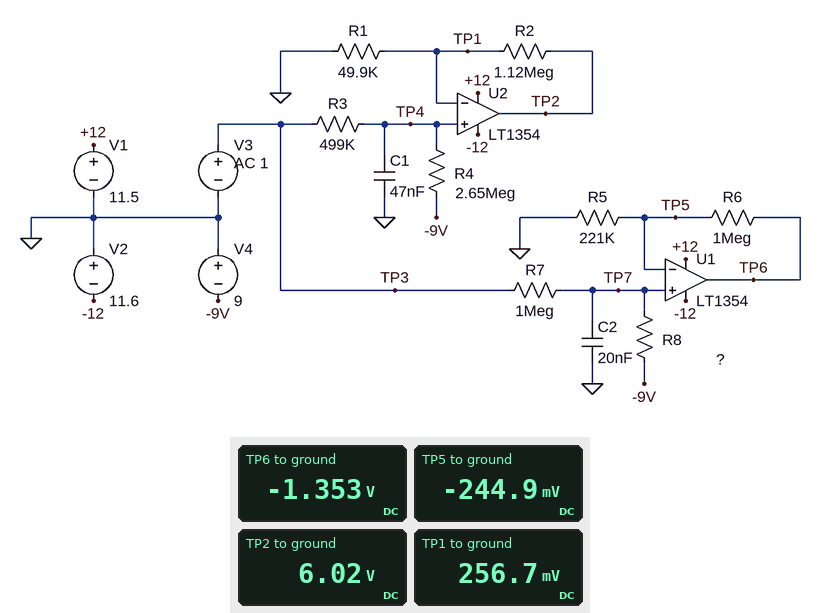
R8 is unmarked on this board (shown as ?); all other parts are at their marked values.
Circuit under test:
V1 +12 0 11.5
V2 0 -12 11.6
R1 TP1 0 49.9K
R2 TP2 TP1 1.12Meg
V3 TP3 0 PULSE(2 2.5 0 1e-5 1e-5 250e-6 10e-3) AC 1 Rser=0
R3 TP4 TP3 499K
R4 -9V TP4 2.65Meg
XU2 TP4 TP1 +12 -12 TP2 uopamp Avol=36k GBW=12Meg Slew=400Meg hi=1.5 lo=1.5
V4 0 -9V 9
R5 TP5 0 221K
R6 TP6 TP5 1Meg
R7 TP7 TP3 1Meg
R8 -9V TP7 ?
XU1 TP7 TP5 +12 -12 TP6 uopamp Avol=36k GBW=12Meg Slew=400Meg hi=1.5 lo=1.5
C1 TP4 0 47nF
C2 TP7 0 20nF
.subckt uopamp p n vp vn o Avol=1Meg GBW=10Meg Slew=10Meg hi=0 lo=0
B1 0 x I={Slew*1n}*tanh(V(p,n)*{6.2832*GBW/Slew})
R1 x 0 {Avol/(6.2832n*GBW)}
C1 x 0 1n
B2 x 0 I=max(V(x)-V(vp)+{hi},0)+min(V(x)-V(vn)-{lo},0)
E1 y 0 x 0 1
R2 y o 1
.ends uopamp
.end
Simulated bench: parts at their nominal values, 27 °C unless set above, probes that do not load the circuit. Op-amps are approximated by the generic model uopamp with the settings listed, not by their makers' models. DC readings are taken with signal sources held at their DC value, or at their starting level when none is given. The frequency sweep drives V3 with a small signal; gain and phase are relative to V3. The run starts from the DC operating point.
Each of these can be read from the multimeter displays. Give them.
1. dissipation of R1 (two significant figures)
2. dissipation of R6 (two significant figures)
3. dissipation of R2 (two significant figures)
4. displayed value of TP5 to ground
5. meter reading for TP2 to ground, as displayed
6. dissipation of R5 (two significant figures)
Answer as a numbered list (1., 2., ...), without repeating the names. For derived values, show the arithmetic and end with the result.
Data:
1. (256.7 mV)^2 / 49.9 kΩ = 1.3 µW
2. (-244.9 mV - (-1.353 V))^2 / 1 MΩ = 1.2 µW
3. (6.02 V - 256.7 mV)^2 / 1.12 MΩ = 30 µW
4. -244.9 mV
5. 6.02 V
6. (0 V - (-244.9 mV))^2 / 221 kΩ = 270 nW
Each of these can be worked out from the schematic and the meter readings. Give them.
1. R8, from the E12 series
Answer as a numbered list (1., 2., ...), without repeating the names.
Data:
1. 3.9 MΩ
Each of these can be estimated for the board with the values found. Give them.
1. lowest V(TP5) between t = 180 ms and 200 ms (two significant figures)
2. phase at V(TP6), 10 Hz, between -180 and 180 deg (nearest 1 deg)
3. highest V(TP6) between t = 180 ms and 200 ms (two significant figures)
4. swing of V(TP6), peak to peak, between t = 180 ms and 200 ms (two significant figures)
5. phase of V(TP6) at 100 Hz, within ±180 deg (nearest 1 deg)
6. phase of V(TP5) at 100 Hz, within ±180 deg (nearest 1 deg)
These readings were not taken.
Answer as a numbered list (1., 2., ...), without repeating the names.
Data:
1. -240 mV
2. -45 deg
3. -1.3 V
4. 35 mV
5. -84 deg
6. -84 deg
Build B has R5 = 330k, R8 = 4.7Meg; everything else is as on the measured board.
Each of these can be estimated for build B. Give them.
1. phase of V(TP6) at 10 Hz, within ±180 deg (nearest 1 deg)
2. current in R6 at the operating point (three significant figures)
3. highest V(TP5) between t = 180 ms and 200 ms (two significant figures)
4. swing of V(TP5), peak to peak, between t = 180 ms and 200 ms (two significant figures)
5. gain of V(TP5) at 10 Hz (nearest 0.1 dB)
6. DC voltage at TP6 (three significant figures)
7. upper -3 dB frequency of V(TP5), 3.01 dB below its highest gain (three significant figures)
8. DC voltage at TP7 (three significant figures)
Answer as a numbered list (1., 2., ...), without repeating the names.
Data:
1. -46 deg
2. 213 nA
3. 84 mV
4. 6.3 mV
5. -4.8 dB
6. 283 mV
7. 9.65 Hz
8. 70.2 mV
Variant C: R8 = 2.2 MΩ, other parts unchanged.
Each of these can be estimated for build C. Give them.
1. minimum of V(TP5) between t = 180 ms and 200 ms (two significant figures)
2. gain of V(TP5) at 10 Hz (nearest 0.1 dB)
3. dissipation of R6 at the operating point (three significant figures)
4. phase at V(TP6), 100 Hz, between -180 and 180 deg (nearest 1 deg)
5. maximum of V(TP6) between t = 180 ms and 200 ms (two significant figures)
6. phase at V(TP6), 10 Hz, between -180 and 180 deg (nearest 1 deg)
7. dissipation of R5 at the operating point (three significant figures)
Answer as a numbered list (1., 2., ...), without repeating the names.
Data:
1. -1.4 V
2. -5.7 dB
3. 42.3 µW
4. -83 deg
5. -7.9 V
6. -41 deg
7. 9.35 µW
